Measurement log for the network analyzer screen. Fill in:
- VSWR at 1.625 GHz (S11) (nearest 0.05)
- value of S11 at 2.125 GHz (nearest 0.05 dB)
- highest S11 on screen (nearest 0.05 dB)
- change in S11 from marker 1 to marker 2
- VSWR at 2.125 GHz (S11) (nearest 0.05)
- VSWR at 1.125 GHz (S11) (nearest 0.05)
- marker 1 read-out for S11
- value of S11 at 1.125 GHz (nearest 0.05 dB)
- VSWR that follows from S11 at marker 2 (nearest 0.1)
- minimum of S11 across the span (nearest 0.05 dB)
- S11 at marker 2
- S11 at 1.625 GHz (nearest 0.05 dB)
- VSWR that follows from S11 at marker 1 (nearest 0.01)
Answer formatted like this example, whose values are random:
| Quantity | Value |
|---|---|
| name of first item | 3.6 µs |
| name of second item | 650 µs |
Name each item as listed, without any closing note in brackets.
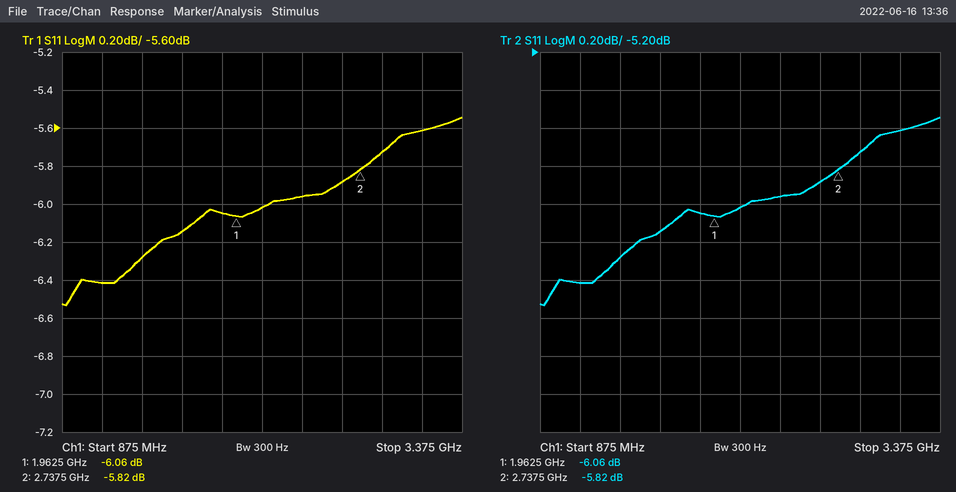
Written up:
| Quantity | Value |
|---|---|
| VSWR at 1.625 GHz (S11) | 2.95 |
| value of S11 at 2.125 GHz | -6.00 dB |
| highest S11 on screen | -5.55 dB |
| change in S11 from marker 1 to marker 2 | 0.24 dB |
| VSWR at 2.125 GHz (S11) | 3.00 |
| VSWR at 1.125 GHz (S11) | 2.85 |
| marker 1 read-out for S11 | -6.06 dB |
| value of S11 at 1.125 GHz | -6.40 dB |
| VSWR that follows from S11 at marker 2 | 3.1 |
| minimum of S11 across the span | -6.55 dB |
| S11 at marker 2 | -5.82 dB |
| S11 at 1.625 GHz | -6.15 dB |
| VSWR that follows from S11 at marker 1 | 2.98 |
